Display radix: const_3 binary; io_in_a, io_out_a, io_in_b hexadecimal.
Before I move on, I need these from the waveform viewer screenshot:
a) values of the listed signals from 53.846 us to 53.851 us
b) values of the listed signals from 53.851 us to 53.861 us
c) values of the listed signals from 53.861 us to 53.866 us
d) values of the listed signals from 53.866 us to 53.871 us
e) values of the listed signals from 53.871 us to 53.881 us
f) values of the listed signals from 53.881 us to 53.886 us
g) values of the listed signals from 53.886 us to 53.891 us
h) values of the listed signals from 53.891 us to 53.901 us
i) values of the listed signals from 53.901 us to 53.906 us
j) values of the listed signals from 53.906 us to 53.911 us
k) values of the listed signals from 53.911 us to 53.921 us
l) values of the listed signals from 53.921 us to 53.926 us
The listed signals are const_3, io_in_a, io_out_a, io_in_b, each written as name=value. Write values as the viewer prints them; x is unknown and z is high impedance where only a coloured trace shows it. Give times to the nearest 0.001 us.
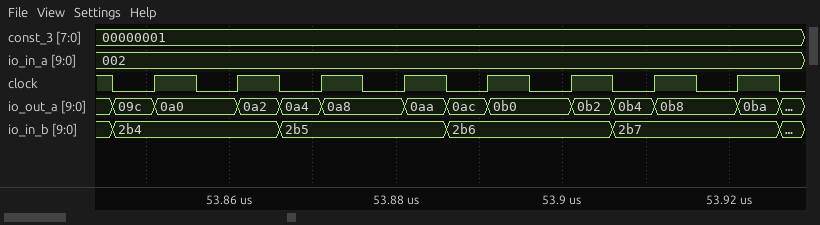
const_3=00000001, io_in_a=002, io_out_a=09c, io_in_b=2b4
const_3=00000001, io_in_a=002, io_out_a=0a0, io_in_b=2b4
const_3=00000001, io_in_a=002, io_out_a=0a2, io_in_b=2b4
const_3=00000001, io_in_a=002, io_out_a=0a4, io_in_b=2b5
const_3=00000001, io_in_a=002, io_out_a=0a8, io_in_b=2b5
const_3=00000001, io_in_a=002, io_out_a=0aa, io_in_b=2b5
const_3=00000001, io_in_a=002, io_out_a=0ac, io_in_b=2b6
const_3=00000001, io_in_a=002, io_out_a=0b0, io_in_b=2b6
const_3=00000001, io_in_a=002, io_out_a=0b2, io_in_b=2b6
const_3=00000001, io_in_a=002, io_out_a=0b4, io_in_b=2b7
const_3=00000001, io_in_a=002, io_out_a=0b8, io_in_b=2b7
const_3=00000001, io_in_a=002, io_out_a=0ba, io_in_b=2b7
